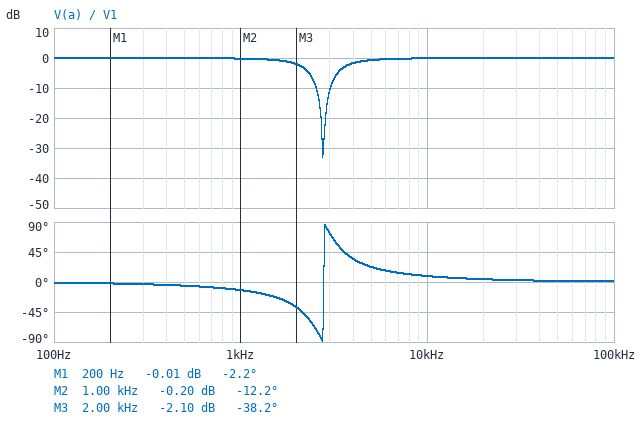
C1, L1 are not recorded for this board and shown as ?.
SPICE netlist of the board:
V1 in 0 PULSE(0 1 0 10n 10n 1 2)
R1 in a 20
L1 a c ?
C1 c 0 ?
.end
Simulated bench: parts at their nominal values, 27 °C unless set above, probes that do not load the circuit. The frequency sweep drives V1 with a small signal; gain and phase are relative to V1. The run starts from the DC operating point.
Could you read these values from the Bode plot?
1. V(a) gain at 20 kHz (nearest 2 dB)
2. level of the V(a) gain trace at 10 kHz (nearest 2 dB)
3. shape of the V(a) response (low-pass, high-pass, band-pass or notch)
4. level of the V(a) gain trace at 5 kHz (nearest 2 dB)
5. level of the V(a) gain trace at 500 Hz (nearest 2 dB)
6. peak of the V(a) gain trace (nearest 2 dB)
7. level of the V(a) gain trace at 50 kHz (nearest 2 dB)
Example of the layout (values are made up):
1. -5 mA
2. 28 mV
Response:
1. 0 dB
2. 0 dB
3. notch
4. 0 dB
5. 0 dB
6. 0 dB
7. 0 dB
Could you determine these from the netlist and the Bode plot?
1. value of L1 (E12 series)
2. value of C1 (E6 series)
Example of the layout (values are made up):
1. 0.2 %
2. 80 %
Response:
1. 2.2 mH
2. 1.5 µF
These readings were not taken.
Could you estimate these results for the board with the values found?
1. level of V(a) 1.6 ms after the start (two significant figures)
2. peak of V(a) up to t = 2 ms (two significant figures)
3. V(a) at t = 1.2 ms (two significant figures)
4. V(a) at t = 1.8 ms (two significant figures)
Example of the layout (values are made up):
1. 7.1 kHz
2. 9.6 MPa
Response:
1. 1.0 V
2. 1.2 V
3. 1.0 V
4. 1.0 V
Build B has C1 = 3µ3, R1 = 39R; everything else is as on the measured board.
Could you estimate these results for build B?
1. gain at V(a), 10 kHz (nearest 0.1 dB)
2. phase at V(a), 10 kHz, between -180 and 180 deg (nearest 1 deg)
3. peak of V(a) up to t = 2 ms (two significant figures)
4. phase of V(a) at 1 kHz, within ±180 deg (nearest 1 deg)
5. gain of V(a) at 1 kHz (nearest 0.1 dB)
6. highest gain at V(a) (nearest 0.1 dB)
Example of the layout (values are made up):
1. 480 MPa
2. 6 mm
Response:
1. -0.4 dB
2. 16 deg
3. 1.0 V
4. -49 deg
5. -3.6 dB
6. 0 dB
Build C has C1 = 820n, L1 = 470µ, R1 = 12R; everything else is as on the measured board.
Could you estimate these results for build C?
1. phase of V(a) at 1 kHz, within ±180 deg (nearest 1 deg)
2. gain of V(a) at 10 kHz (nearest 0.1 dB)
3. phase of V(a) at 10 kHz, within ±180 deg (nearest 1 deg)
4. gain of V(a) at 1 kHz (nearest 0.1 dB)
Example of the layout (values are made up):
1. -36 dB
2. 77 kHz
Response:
1. -4 deg
2. -3.8 dB
3. 50 deg
4. 0 dB
